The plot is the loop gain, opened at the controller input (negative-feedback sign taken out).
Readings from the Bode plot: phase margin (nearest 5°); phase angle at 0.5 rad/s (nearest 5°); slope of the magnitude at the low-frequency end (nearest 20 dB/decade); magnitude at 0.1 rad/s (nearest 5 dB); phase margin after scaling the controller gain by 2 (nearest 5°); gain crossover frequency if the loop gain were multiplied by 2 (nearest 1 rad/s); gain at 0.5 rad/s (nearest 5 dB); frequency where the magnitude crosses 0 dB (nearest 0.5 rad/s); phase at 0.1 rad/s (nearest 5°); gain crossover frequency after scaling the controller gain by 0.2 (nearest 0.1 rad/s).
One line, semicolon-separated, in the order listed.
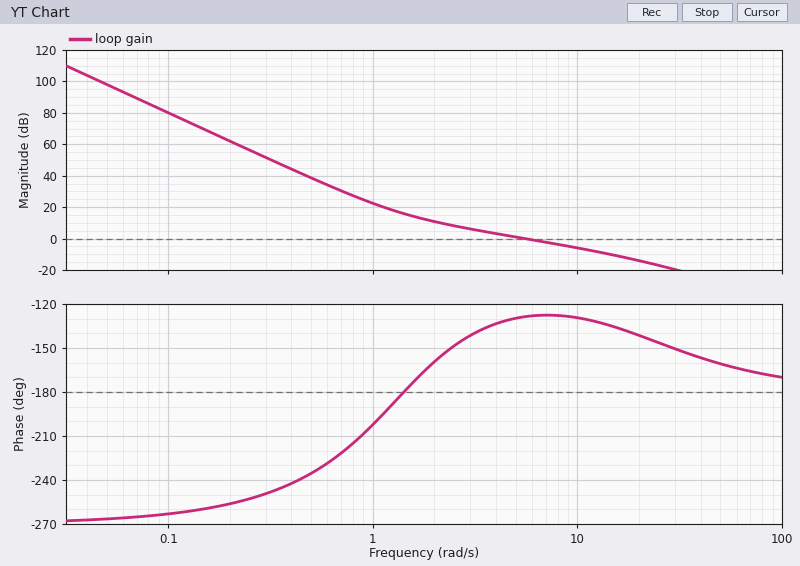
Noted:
50°; -235°; -60 dB/decade; 80 dB; 50°; 10 rad/s; 40 dB; 5.5 rad/s; -265°; 1.6 rad/s
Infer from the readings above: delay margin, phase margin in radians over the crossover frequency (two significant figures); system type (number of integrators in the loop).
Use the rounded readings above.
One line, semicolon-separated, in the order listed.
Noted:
0.16 s; 3
